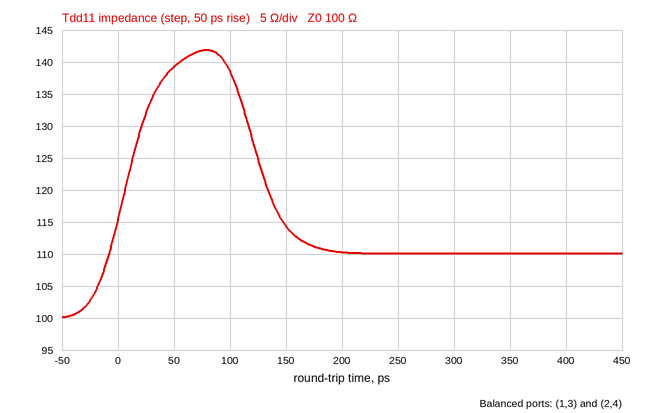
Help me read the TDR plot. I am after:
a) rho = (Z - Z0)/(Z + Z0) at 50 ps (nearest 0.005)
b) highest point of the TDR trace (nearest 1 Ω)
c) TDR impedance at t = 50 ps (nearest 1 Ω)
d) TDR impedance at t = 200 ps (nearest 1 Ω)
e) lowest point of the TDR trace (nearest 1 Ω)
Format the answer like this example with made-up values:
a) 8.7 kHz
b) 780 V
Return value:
a) +0.165
b) 142 Ω
c) 139 Ω
d) 110 Ω
e) 100 Ω
